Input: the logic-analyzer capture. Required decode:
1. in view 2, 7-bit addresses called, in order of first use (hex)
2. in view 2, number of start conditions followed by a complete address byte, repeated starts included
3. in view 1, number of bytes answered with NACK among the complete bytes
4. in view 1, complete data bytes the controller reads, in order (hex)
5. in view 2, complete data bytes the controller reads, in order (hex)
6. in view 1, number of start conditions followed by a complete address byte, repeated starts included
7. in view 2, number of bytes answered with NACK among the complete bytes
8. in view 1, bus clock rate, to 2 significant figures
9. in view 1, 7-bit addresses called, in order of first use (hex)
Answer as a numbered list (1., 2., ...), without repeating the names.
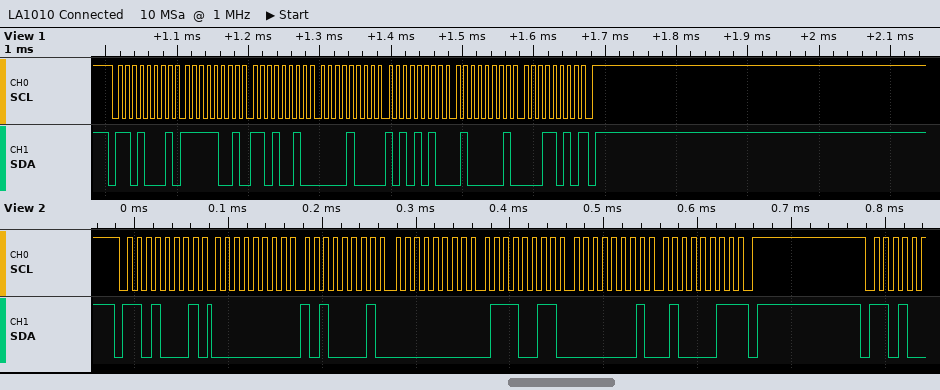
1. 0x68
2. 1
3. 1
4. F9 D2 08 AA 41 1A
5. 00 A1 00 73 01 43
6. 1
7. 1
8. 100 kHz
9. 0x68
